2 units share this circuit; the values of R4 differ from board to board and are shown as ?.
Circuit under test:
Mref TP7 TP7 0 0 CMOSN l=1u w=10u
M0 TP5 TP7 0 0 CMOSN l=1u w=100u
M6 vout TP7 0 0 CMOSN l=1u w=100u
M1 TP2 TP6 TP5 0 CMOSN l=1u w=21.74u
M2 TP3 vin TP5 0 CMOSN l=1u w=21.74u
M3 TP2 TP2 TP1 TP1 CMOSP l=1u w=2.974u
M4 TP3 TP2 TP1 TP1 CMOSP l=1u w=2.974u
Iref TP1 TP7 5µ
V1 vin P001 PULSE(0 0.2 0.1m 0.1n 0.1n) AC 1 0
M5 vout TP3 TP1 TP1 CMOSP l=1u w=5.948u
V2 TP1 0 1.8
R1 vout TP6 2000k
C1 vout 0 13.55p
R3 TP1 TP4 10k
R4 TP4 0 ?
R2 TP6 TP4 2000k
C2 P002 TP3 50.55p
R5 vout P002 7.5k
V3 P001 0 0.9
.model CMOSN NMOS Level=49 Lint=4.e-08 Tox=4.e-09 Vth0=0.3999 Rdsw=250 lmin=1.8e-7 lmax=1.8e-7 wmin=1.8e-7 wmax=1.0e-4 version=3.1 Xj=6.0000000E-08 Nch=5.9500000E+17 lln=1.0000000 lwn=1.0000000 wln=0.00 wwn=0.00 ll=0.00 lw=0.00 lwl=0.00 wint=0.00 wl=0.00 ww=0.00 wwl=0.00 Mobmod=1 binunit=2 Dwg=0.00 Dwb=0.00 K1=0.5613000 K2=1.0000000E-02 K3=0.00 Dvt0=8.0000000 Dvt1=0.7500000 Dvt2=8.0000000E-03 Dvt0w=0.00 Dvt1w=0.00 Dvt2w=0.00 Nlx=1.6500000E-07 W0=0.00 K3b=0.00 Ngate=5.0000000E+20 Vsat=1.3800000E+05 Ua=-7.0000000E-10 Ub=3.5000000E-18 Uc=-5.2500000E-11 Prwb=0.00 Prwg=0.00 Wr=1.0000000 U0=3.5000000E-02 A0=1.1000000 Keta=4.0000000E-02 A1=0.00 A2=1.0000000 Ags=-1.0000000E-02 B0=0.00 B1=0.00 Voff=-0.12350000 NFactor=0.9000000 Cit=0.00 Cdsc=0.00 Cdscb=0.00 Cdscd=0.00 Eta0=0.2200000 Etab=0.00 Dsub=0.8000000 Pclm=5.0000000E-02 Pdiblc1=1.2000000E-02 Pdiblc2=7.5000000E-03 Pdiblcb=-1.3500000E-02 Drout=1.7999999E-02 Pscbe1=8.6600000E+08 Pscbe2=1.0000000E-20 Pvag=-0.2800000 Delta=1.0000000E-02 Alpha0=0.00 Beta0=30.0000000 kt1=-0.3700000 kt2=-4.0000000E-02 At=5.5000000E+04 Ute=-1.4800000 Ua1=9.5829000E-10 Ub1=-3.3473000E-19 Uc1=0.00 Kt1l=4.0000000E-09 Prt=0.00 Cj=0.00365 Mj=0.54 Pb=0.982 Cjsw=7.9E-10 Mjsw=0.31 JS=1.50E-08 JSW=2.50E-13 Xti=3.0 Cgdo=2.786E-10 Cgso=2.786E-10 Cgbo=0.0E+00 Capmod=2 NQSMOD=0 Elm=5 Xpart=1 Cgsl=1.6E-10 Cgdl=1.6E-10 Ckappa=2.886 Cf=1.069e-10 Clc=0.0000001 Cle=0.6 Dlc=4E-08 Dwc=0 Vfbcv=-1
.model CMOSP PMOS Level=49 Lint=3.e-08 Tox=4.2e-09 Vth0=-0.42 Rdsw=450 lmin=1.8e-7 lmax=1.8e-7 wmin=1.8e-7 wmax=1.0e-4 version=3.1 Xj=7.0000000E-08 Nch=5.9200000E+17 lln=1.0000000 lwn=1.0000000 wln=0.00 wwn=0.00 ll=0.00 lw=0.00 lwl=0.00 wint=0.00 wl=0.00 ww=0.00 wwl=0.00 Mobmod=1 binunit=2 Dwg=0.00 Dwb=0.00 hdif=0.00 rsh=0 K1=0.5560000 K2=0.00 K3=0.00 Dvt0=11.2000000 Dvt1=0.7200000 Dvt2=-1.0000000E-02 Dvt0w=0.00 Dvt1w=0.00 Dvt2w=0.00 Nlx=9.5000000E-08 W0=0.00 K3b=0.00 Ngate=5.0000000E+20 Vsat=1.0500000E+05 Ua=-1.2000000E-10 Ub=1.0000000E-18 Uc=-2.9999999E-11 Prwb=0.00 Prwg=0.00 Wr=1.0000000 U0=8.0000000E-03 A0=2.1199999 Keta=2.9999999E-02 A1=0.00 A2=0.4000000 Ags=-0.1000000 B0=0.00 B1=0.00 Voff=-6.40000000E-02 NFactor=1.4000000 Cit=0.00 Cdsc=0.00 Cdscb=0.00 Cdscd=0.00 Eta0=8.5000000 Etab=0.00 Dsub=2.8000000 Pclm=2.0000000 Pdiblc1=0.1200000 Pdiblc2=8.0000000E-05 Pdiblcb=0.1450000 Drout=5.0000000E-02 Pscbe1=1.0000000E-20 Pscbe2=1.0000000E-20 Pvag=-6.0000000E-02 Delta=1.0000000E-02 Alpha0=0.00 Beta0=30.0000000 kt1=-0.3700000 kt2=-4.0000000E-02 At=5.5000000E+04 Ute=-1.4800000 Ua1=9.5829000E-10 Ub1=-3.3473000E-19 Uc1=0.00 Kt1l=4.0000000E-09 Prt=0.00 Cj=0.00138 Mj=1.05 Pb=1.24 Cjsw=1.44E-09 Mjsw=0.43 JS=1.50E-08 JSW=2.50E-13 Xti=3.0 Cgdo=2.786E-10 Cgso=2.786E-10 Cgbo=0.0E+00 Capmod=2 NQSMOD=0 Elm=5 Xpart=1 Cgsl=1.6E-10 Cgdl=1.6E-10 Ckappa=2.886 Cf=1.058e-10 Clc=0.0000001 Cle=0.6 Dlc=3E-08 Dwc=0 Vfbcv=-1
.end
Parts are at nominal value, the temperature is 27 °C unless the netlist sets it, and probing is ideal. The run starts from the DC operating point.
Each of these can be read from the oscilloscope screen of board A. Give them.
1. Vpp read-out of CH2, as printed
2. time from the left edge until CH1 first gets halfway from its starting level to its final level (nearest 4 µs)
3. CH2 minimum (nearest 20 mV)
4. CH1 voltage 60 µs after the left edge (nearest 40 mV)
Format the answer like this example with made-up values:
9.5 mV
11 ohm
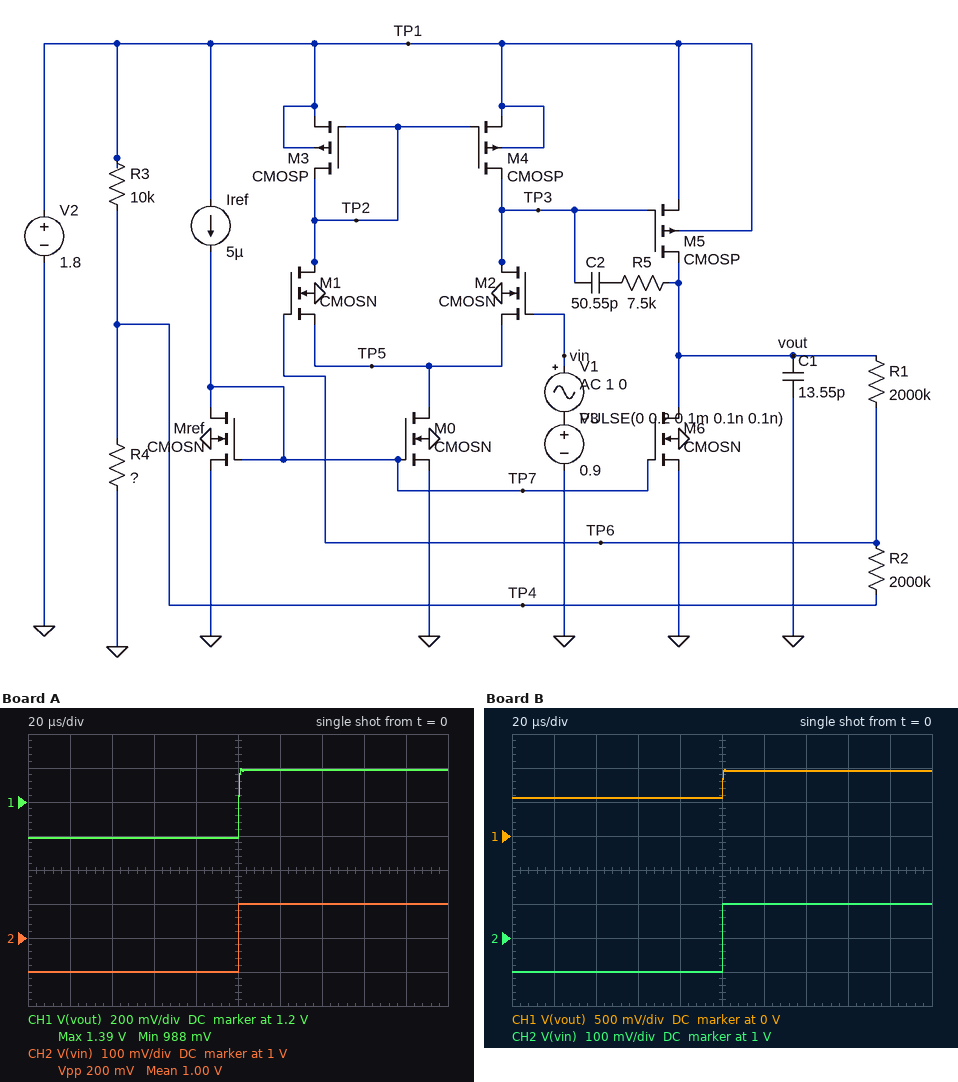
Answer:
200 mV
100 µs
900 mV
1.00 V
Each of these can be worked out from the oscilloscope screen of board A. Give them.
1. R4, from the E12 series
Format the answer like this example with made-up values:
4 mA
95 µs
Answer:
8.2 kΩ
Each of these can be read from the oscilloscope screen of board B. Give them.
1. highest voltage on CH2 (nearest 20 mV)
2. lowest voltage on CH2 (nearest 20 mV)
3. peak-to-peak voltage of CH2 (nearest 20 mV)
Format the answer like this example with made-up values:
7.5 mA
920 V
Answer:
1.10 V
900 mV
200 mV
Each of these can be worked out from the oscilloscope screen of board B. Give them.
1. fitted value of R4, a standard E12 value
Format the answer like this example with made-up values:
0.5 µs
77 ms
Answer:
22 kΩ
